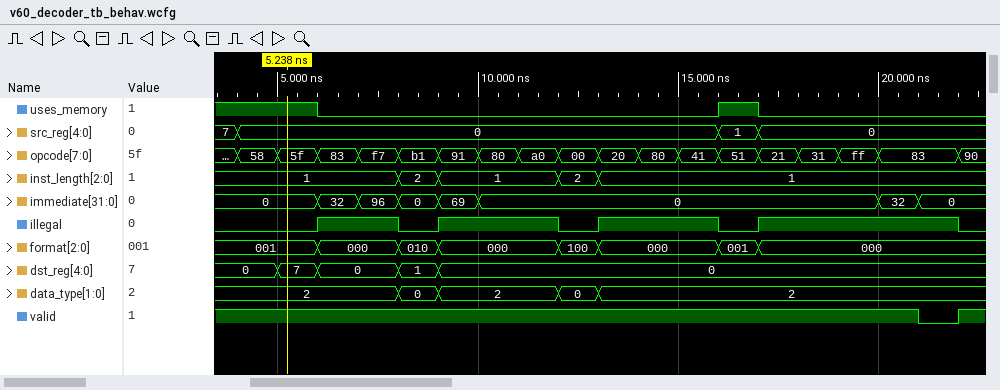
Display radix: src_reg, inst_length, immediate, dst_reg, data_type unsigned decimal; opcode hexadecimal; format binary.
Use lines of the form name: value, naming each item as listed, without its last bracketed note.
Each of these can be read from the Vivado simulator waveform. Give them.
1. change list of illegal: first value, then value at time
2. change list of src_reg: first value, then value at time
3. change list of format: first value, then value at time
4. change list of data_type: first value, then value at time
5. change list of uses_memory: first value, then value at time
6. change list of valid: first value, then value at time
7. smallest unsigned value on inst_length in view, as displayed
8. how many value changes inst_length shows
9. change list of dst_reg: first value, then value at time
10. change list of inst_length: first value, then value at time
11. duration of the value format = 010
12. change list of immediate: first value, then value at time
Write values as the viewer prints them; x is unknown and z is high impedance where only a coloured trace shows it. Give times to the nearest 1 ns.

change list of illegal: first value, then value at time: 0, 1 at 6 ns, 0 at 8 ns, 1 at 9 ns, 0 at 12 ns, 1 at 13 ns, 0 at 16 ns, 1 at 17 ns, 0 at 22 ns
change list of src_reg: first value, then value at time: 7, 0 at 4 ns, 1 at 16 ns, 0 at 17 ns
change list of format: first value, then value at time: 001, 000 at 6 ns, 010 at 8 ns, 000 at 9 ns, 100 at 12 ns, 000 at 13 ns, 001 at 16 ns, 000 at 17 ns
change list of data_type: first value, then value at time: 2, 0 at 8 ns, 2 at 9 ns, 0 at 12 ns, 2 at 13 ns
change list of uses_memory: first value, then value at time: 1, 0 at 6 ns, 1 at 16 ns, 0 at 17 ns
change list of valid: first value, then value at time: 1, 0 at 21 ns, 1 at 22 ns
smallest unsigned value on inst_length in view, as displayed: 1
how many value changes inst_length shows: 4
change list of dst_reg: first value, then value at time: 0, 7 at 5 ns, 0 at 6 ns, 1 at 8 ns, 0 at 9 ns
change list of inst_length: first value, then value at time: 1, 2 at 8 ns, 1 at 9 ns, 2 at 12 ns, 1 at 13 ns
duration of the value format = 010: 1 ns
change list of immediate: first value, then value at time: 0, 32 at 6 ns, 96 at 7 ns, 0 at 8 ns, 69 at 9 ns, 0 at 10 ns, 32 at 20 ns, 0 at 21 ns
